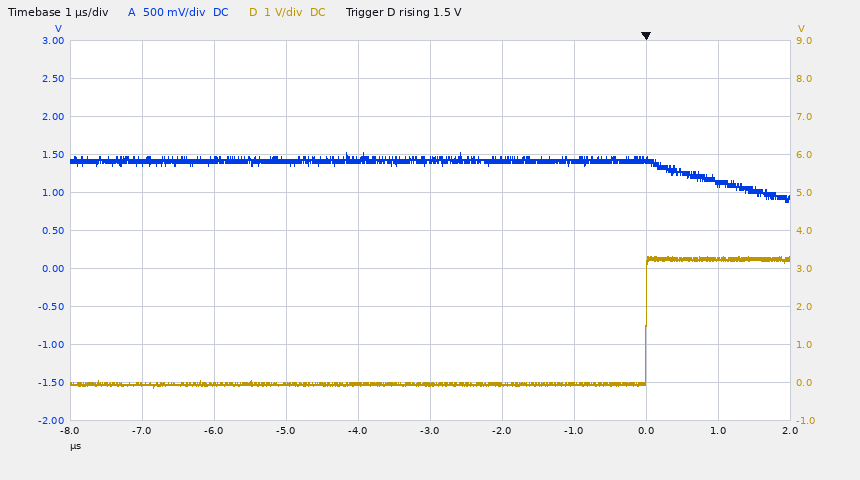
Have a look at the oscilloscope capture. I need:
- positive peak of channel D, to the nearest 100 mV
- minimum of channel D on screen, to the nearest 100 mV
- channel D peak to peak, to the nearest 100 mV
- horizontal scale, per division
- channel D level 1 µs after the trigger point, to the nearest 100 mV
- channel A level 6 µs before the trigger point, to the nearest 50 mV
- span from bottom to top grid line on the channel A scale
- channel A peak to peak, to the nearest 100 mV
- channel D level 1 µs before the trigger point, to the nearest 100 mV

3.3 V
-100 mV
3.4 V
1 µs
3.2 V
1.45 V
5 V
600 mV
0.0 V
